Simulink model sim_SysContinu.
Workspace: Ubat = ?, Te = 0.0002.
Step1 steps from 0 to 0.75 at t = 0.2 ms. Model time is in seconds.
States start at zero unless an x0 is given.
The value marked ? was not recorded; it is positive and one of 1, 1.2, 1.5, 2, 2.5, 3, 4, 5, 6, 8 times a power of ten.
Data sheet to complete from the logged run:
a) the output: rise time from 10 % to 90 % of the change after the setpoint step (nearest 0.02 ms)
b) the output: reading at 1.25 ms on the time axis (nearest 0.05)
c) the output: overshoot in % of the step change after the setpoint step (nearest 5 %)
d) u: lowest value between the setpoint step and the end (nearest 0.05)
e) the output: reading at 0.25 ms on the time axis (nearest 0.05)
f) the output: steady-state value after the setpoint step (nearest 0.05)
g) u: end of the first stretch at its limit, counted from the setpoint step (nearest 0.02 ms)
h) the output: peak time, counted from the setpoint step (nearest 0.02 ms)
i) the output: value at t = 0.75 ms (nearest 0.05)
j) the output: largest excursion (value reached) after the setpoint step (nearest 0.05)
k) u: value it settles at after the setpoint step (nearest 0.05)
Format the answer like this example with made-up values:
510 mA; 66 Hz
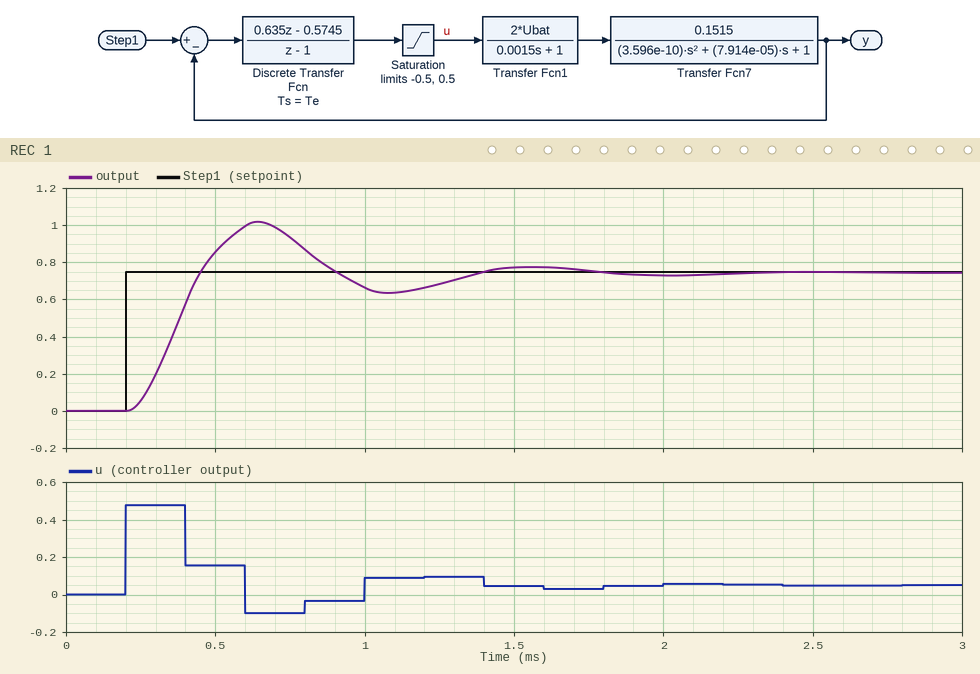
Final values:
0.16 ms; 0.70; 35 %; -0.10; 0.05; 0.75; 0.20 ms; 0.44 ms; 0.95; 1.00; 0.05
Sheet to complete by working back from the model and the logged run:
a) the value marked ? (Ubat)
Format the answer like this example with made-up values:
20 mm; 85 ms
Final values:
50
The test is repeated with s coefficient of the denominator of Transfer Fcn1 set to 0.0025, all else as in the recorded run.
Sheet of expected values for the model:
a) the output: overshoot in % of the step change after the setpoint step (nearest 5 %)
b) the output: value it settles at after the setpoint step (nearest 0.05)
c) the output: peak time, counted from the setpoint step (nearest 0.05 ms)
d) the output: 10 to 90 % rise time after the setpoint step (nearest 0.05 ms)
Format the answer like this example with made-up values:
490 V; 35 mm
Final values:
15 %; 0.75; 0.65 ms; 0.30 ms
